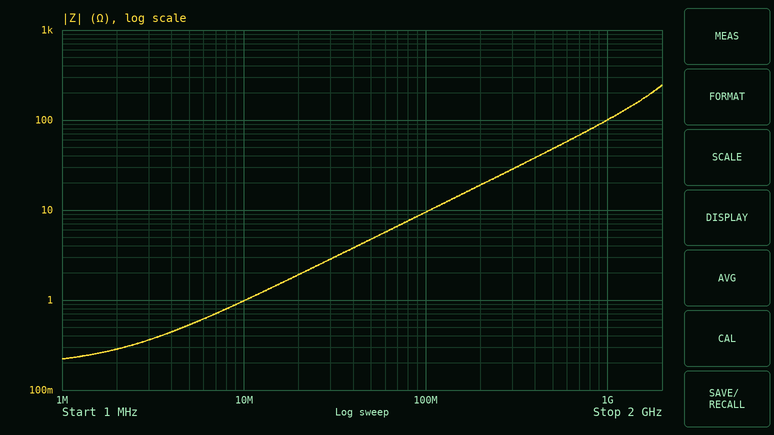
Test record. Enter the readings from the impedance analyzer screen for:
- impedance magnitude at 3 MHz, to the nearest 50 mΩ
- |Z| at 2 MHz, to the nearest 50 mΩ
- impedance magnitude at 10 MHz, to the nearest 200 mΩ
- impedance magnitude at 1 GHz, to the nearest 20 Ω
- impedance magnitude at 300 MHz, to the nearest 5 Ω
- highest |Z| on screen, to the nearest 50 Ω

350 mΩ
300 mΩ
1.0 Ω
100 Ω
30 Ω
250 Ω
